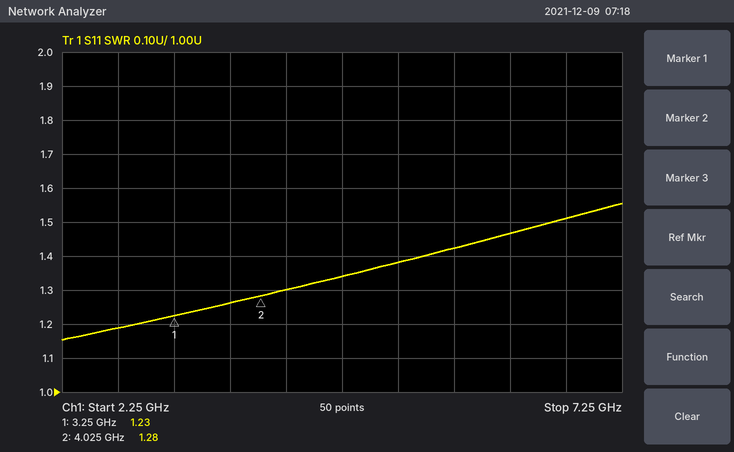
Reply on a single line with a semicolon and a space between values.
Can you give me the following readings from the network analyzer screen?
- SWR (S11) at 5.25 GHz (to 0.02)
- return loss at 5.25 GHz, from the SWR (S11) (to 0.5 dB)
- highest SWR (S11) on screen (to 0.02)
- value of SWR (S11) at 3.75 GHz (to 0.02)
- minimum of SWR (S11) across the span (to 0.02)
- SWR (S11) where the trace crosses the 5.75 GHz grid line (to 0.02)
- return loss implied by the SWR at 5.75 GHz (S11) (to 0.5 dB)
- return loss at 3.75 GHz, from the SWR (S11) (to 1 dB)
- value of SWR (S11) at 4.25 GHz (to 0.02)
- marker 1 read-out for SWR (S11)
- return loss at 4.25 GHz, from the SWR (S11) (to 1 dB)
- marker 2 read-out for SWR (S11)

1.38; 16.0 dB; 1.56; 1.26; 1.16; 1.42; 15.0 dB; 19 dB; 1.30; 1.23; 18 dB; 1.28
